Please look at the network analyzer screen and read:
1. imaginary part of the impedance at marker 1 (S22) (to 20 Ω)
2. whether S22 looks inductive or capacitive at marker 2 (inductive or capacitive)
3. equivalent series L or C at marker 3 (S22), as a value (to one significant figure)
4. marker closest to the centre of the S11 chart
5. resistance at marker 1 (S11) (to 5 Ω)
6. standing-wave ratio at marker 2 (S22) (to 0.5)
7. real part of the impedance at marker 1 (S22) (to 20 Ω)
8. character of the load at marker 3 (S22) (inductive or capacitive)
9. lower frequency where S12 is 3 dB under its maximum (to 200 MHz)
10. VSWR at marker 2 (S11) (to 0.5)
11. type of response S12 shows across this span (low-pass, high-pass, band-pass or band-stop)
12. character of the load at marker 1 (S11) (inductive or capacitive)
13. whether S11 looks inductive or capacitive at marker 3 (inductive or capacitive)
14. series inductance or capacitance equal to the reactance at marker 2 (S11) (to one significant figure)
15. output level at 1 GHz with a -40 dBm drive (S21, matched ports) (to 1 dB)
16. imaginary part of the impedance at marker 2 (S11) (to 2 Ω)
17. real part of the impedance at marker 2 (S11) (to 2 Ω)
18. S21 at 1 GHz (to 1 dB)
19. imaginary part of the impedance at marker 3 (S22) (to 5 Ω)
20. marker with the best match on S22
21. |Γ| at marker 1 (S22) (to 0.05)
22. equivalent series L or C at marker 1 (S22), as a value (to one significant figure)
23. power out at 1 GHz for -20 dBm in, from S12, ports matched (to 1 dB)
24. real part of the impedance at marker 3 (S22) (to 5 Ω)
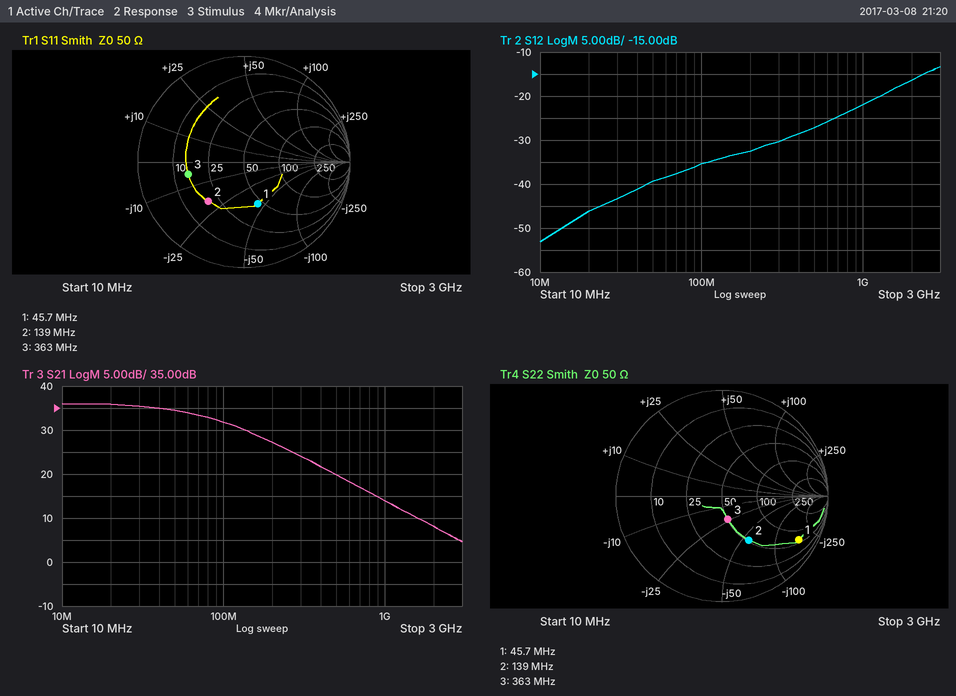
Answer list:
-160 Ω
capacitive
20 pF
marker 1
45 Ω
3.0
60 Ω
capacitive
2.0 GHz
3.0
high-pass
capacitive
capacitive
60 pF
-26 dBm
-20 Ω
20 Ω
14 dB
-25 Ω
marker 3
0.85
20 pF
-42 dBm
50 Ω
